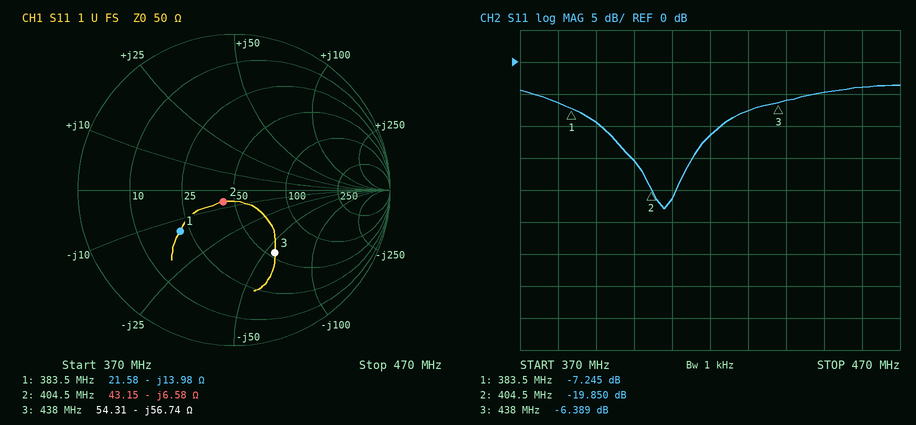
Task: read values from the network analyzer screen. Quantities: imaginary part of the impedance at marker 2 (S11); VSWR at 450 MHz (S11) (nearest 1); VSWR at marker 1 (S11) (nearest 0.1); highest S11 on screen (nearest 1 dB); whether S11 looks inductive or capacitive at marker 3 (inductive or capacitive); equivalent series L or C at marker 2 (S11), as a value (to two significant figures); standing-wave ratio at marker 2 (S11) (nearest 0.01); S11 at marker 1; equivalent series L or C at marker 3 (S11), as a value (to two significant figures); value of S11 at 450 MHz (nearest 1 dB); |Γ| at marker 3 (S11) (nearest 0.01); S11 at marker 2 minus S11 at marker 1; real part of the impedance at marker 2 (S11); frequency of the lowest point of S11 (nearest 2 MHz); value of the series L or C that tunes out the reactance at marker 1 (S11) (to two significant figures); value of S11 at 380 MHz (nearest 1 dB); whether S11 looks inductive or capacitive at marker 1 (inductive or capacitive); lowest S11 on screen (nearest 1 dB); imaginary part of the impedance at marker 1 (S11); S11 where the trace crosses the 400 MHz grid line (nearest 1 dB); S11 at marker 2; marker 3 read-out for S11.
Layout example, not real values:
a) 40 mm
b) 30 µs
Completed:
a) -6.58 Ω
b) 4
c) 2.5
d) -4 dB
e) capacitive
f) 60 pF
g) 1.23
h) -7.245 dB
i) 6.4 pF
j) -5 dB
k) 0.48
l) -12.605 dB
m) 43.15 Ω
n) 408 MHz
o) 5.8 nH
p) -6 dB
q) capacitive
r) -23 dB
s) -13.98 Ω
t) -15 dB
u) -19.850 dB
v) -6.389 dB
